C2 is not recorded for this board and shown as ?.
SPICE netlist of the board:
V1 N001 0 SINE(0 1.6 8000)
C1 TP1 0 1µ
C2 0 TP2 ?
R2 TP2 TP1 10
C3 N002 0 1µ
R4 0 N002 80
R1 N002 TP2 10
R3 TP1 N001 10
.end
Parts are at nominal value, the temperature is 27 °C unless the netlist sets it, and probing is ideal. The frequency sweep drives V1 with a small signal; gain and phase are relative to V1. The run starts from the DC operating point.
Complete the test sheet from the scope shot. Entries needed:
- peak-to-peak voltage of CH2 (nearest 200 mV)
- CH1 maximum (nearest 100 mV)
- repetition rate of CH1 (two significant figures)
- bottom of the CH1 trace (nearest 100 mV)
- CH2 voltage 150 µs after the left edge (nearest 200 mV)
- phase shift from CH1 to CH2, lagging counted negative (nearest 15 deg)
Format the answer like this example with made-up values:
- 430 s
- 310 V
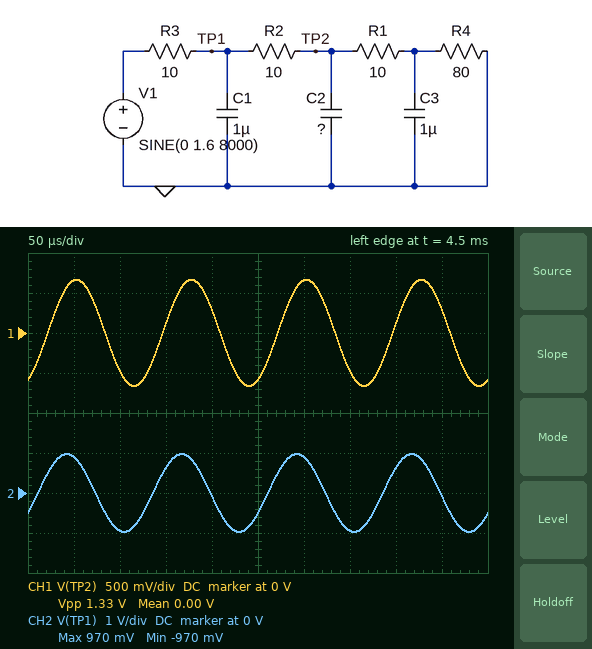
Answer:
- 2.0 V
- 700 mV
- 8.0 kHz
- -700 mV
- 600 mV
- 30 deg
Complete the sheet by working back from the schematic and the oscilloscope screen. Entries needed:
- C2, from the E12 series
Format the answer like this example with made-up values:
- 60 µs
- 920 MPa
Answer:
- 820 nF
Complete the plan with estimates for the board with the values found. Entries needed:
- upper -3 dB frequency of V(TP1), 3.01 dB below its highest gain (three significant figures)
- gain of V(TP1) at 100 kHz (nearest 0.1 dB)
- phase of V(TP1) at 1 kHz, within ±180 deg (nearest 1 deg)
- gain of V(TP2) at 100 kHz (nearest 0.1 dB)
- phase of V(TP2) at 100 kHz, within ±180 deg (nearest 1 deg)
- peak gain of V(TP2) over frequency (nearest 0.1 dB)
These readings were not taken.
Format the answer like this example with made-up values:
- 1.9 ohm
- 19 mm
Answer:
- 6.73 kHz
- -16.6 dB
- -7 deg
- -31.6 dB
- -143 deg
- -1.7 dB
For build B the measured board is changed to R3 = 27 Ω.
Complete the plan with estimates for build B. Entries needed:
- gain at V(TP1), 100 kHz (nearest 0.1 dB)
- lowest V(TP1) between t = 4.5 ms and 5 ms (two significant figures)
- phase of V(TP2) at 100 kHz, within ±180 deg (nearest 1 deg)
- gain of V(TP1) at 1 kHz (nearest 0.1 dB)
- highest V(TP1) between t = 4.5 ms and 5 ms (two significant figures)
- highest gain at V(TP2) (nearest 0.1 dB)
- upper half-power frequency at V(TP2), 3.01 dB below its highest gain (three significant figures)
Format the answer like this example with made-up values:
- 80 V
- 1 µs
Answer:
- -25.0 dB
- -510 mV
- -148 deg
- -2.6 dB
- 510 mV
- -3.0 dB
- 2.59 kHz
